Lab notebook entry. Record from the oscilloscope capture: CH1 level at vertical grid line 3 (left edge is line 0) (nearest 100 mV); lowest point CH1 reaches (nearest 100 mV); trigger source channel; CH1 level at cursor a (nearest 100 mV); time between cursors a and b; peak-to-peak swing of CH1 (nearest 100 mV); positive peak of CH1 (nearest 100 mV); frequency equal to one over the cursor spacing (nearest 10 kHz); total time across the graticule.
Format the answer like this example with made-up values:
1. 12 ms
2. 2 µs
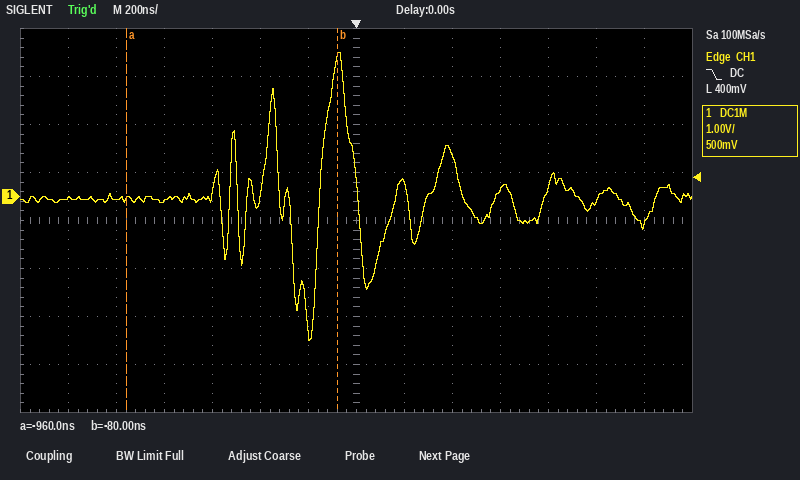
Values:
1. -100 mV
2. -3.0 V
3. CH1
4. -100 mV
5. 880 ns
6. 6.0 V
7. 3.0 V
8. 1.14 MHz
9. 2.8 µs
